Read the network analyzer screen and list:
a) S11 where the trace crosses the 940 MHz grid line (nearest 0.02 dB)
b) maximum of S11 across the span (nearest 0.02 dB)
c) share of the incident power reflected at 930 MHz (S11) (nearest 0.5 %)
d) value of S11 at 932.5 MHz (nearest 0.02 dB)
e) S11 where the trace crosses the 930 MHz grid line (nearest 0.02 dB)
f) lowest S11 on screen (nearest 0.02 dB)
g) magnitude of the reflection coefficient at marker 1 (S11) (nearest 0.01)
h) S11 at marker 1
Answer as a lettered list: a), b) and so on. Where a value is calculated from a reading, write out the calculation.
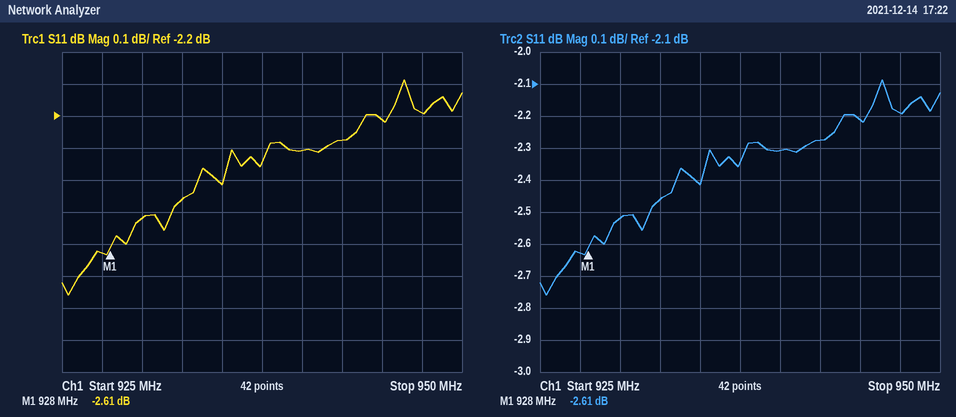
a) -2.30 dB
b) -2.08 dB
c) 10^(-2.52/10) ≈ 56.0 %
d) -2.46 dB
e) -2.52 dB
f) -2.76 dB
g) 10^(-2.61/20) ≈ 0.74
h) -2.61 dB
